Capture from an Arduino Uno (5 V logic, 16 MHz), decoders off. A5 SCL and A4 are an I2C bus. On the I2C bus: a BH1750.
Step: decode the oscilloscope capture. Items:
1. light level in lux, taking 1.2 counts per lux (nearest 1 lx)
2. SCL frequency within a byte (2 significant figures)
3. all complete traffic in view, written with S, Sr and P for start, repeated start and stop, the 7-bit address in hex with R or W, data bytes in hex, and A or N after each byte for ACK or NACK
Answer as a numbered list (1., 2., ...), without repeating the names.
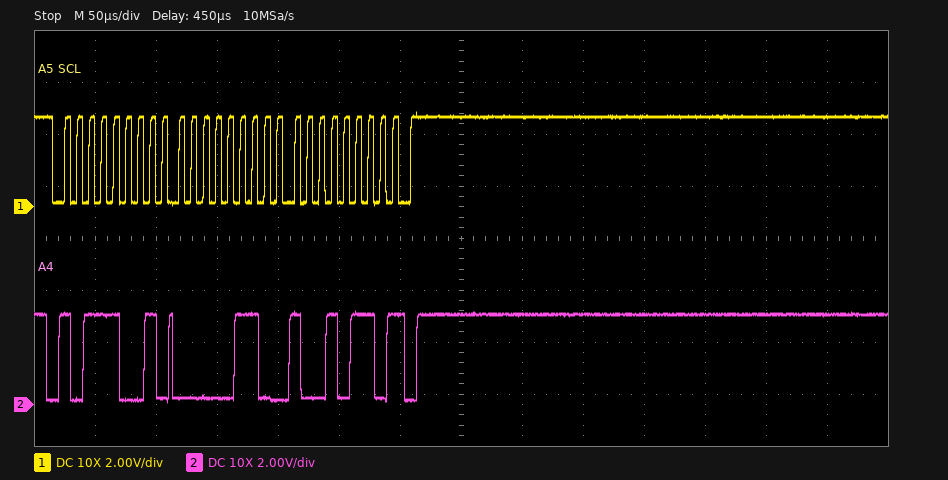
1. 1405 lx
2. 100 kHz
3. S 5CR A 06 A 96 N P
